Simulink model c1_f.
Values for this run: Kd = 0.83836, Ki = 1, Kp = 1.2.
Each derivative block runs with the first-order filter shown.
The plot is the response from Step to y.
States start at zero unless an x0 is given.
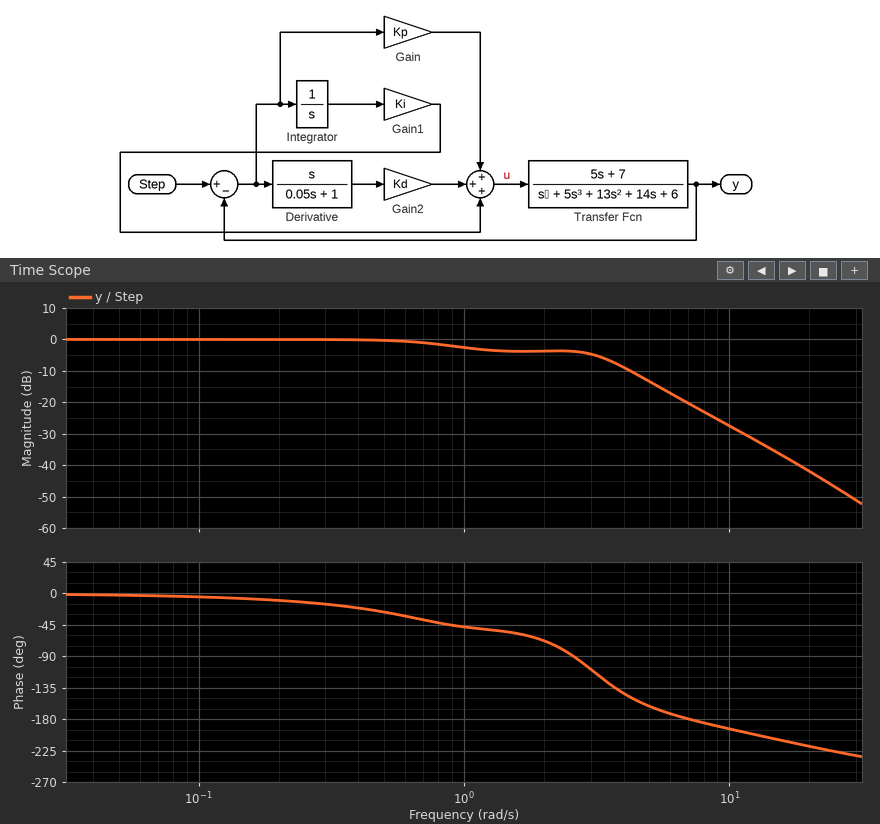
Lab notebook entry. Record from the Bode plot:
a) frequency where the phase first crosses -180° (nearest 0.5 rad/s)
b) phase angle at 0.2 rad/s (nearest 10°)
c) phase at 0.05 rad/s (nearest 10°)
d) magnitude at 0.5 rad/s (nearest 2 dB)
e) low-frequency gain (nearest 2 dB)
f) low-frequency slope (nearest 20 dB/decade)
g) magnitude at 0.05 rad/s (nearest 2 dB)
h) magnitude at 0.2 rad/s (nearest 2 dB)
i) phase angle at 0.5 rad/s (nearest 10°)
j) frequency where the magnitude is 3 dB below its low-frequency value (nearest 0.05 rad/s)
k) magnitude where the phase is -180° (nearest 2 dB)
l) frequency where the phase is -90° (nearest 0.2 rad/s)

7.0 rad/s
-10°
0°
0 dB
0 dB
0 dB/decade
0 dB
0 dB
-30°
1.10 rad/s
-20 dB
2.6 rad/s
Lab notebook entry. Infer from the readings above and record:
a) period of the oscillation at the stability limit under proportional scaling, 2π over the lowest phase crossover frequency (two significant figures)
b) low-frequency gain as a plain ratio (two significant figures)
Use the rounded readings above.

0.90 s
1.0
